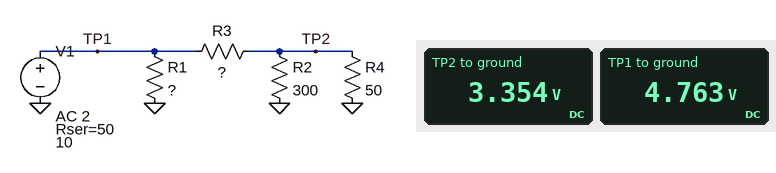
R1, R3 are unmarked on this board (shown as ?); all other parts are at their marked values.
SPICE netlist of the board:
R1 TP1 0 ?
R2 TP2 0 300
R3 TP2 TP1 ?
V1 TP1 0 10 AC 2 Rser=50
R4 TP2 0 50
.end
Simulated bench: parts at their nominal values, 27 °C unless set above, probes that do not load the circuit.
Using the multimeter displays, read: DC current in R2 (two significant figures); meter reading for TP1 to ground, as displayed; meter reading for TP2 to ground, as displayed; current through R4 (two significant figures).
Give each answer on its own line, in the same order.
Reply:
11 mA
4.763 V
3.354 V
67 mA
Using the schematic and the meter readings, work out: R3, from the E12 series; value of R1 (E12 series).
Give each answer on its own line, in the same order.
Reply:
18 Ω
180 Ω
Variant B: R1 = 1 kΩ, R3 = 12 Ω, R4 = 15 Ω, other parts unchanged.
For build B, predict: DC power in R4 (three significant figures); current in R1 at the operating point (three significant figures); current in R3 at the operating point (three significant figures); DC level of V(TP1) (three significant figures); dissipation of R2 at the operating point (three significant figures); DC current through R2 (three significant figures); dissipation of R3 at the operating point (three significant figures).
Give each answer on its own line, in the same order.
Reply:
226 mW
3.39 mA
129 mA
3.39 V
11.3 mW
6.14 mA
199 mW
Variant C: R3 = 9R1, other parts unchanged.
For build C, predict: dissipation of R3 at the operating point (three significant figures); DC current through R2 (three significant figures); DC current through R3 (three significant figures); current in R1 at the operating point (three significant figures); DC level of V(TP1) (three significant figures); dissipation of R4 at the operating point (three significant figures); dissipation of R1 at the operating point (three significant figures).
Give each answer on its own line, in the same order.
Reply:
67.2 mW
12.3 mA
85.9 mA
24.8 mA
4.46 V
271 mW
111 mW
